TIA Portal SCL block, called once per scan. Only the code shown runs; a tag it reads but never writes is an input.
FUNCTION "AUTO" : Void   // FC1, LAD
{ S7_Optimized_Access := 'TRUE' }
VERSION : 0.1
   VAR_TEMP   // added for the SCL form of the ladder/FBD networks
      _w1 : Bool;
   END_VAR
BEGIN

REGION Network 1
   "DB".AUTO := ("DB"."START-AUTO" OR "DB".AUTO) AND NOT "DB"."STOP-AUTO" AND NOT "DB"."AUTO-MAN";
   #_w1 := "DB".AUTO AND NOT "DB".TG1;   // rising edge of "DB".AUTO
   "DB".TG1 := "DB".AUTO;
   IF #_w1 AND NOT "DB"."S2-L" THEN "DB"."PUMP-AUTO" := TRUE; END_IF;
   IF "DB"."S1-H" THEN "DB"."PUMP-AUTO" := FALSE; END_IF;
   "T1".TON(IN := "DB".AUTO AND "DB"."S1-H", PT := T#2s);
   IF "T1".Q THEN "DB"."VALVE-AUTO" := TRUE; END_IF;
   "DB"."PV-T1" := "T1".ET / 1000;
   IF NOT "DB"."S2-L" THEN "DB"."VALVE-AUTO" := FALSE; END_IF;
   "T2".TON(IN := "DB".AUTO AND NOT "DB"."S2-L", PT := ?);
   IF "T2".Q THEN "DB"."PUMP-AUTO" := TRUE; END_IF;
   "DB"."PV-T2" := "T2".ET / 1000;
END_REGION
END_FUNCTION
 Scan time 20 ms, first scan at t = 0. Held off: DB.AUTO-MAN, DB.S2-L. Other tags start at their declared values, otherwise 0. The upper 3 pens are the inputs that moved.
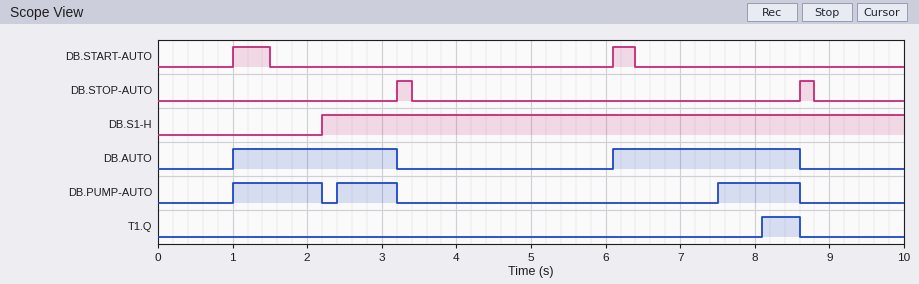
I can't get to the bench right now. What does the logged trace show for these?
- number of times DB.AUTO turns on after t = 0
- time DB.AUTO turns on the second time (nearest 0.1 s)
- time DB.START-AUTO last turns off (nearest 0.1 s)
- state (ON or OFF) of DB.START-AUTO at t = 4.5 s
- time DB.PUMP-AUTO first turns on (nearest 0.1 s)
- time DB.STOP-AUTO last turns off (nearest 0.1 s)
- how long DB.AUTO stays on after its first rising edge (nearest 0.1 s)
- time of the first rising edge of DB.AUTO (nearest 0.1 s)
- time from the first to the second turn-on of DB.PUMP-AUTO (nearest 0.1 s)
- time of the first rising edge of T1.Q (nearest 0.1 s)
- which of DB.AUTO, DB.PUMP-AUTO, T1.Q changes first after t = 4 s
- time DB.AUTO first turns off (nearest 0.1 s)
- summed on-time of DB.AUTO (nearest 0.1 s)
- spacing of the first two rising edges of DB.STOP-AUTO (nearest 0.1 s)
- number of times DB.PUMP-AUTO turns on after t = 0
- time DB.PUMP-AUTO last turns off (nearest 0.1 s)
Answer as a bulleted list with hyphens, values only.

- 2
- 6.1 s
- 6.4 s
- OFF
- 1.0 s
- 8.8 s
- 2.2 s
- 1.0 s
- 1.4 s
- 8.1 s
- DB.AUTO
- 3.2 s
- 4.7 s
- 5.4 s
- 3
- 8.6 s
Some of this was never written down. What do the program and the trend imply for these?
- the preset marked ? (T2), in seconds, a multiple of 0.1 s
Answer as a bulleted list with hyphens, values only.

- 1.4 s
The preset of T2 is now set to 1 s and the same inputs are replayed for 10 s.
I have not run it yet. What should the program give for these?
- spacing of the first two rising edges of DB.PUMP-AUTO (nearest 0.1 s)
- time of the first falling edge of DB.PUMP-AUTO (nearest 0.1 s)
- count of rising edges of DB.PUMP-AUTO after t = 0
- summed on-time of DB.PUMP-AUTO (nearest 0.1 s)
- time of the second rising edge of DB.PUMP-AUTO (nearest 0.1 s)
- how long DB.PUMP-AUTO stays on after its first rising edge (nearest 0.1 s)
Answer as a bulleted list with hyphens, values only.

- 6.1 s
- 3.2 s
- 2
- 3.7 s
- 7.1 s
- 2.2 s
